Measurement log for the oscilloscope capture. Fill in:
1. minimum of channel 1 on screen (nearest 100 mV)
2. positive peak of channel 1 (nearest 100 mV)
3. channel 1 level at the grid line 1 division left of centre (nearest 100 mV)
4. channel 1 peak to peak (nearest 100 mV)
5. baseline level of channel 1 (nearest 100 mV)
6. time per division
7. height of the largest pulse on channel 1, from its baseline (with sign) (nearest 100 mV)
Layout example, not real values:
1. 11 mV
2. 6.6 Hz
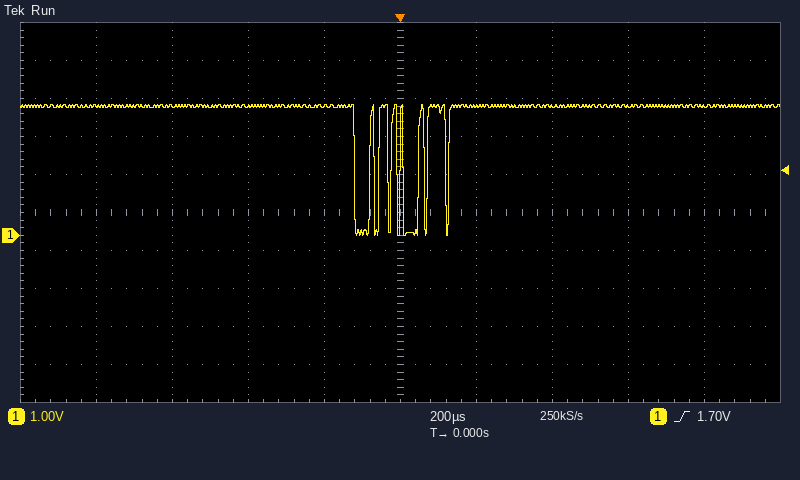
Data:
1. 0.0 V
2. 3.4 V
3. 3.4 V
4. 3.4 V
5. 3.4 V
6. 200 µs
7. -3.4 V
